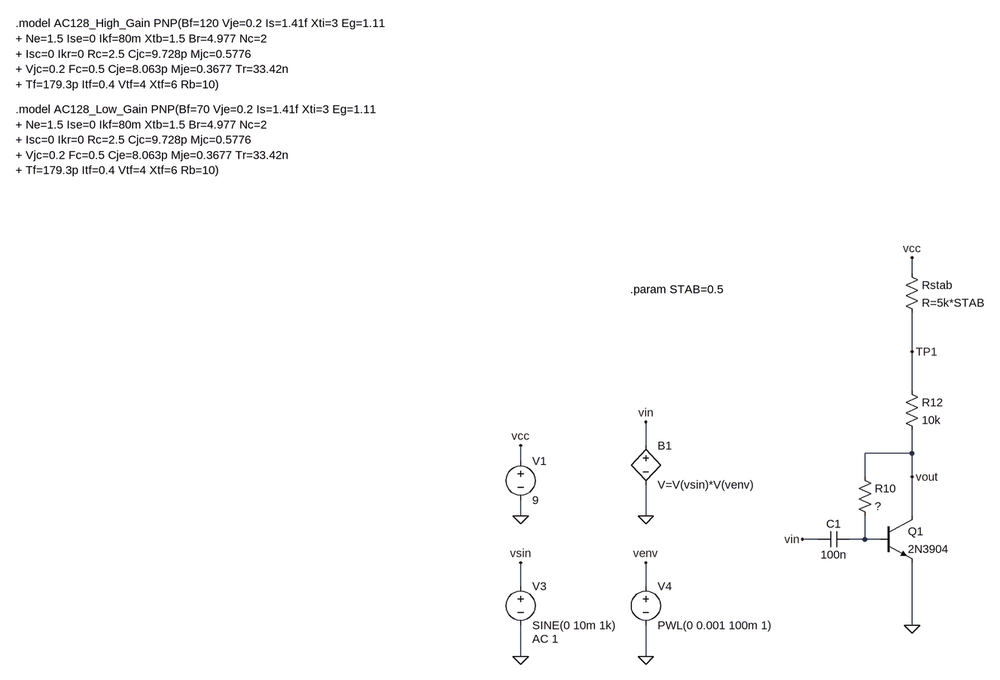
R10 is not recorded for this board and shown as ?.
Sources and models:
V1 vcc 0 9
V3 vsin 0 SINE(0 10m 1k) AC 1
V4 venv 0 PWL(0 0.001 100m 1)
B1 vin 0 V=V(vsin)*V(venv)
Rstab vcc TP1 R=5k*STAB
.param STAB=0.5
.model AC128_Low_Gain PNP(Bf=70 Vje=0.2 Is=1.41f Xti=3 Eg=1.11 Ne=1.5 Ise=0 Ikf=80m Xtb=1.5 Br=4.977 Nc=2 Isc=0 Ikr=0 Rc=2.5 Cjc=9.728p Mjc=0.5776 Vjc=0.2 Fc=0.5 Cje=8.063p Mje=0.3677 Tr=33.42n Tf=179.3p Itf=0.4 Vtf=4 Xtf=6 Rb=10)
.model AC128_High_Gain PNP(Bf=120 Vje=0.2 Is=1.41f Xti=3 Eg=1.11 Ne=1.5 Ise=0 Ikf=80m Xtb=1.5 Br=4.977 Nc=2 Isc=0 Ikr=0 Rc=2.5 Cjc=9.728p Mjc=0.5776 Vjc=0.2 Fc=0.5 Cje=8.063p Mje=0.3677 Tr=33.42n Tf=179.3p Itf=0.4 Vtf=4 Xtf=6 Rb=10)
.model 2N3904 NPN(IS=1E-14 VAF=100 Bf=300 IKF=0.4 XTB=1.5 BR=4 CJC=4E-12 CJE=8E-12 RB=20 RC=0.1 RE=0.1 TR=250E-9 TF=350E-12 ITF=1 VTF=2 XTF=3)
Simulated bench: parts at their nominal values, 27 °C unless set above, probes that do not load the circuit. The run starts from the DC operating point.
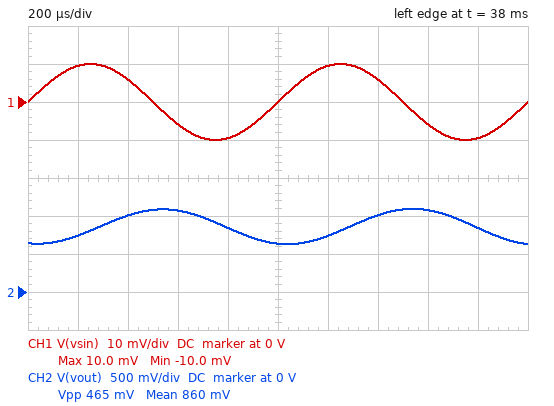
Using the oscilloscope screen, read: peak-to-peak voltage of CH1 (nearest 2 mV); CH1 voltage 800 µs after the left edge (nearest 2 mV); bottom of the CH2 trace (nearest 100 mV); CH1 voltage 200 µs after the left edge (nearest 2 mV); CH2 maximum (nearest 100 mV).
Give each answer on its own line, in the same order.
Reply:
20 mV
-10 mV
600 mV
10 mV
1.1 V
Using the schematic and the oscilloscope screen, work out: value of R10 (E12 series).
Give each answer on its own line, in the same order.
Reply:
100 kΩ
